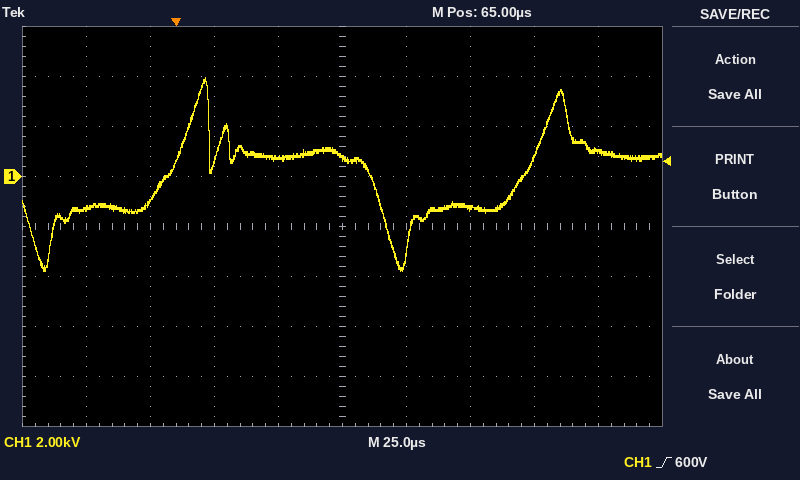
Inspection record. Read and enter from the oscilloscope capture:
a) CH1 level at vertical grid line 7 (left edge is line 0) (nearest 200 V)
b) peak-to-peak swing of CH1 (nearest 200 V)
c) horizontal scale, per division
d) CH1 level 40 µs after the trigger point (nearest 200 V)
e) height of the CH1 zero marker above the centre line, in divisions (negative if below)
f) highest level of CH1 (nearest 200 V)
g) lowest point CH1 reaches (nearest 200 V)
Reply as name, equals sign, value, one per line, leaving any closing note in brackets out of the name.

CH1 level at vertical grid line 7 (left edge is line 0) = -1.2 kV
peak-to-peak swing of CH1 = 7.8 kV
horizontal scale, per division = 25 µs
CH1 level 40 µs after the trigger point = 800 V
height of the CH1 zero marker above the centre line, in divisions = +1.0 div
highest level of CH1 = 4.0 kV
lowest point CH1 reaches = -3.8 kV
